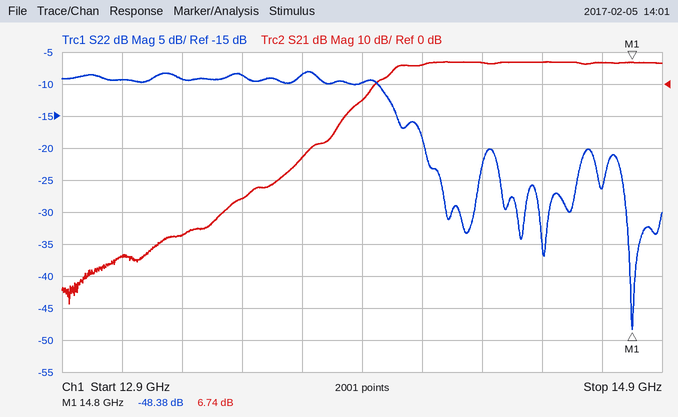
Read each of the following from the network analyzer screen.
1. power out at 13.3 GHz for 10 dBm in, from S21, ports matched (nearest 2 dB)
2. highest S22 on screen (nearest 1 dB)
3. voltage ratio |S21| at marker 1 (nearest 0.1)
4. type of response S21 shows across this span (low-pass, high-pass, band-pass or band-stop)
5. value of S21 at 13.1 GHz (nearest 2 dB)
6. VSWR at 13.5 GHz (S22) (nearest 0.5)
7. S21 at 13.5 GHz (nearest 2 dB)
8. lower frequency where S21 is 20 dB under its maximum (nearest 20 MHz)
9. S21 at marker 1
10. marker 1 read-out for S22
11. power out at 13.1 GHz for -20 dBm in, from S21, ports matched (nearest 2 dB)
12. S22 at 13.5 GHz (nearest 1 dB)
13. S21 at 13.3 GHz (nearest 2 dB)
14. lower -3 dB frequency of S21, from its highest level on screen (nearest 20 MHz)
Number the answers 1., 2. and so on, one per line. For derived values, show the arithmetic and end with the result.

1. 10 dBm + (-48 dB) = -38 dBm
2. -8 dB
3. 10^(6.74/20) ≈ 2.2
4. high-pass
5. -54 dB
6. |Γ| = 10^(-9/20) = 0.3548; VSWR = (1 + 0.3548)/(1 − 0.3548) ≈ 2.10, so 2.0 to the nearest 0.5
7. -36 dB
8. 13.82 GHz
9. 6.74 dB
10. -48.38 dB
11. -20 dBm + (-54 dB) = -74 dBm
12. -9 dB
13. -48 dB
14. 14.00 GHz
